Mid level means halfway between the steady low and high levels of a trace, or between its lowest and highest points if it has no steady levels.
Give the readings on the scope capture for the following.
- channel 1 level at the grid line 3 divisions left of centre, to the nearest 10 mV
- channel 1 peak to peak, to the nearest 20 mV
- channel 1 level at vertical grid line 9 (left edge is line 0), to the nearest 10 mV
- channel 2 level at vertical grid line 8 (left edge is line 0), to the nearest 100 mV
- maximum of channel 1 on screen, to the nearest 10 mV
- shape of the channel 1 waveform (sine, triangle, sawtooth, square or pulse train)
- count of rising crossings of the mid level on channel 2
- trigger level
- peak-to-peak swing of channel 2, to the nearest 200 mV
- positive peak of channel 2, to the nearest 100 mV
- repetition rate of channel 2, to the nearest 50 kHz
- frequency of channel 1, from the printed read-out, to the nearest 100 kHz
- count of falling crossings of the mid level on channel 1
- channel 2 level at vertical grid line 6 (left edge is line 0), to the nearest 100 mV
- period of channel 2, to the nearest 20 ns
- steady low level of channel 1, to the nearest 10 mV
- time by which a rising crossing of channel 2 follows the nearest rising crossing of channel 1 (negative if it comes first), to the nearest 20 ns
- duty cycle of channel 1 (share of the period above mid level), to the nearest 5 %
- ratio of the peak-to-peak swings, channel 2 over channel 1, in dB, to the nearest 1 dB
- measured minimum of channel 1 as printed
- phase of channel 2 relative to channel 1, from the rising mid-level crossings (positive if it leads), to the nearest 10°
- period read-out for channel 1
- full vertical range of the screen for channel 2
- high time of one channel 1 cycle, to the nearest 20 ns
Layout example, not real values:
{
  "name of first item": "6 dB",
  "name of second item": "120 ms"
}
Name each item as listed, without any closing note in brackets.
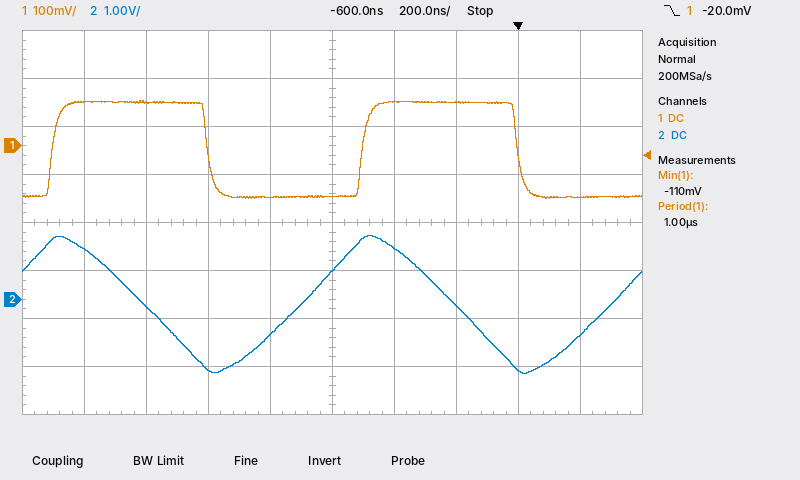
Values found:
{
  "channel 1 level at the grid line 3 divisions left of centre, to the nearest 10 mV": "90 mV",
  "channel 1 peak to peak, to the nearest 20 mV": "200 mV",
  "channel 1 level at vertical grid line 9 (left edge is line 0), to the nearest 10 mV": "-110 mV",
  "channel 2 level at vertical grid line 8 (left edge is line 0), to the nearest 100 mV": "-1.5 V",
  "maximum of channel 1 on screen, to the nearest 10 mV": "90 mV",
  "shape of the channel 1 waveform": "square",
  "count of rising crossings of the mid level on channel 2": "2",
  "trigger level": "-20.0 mV",
  "peak-to-peak swing of channel 2, to the nearest 200 mV": "2.8 V",
  "positive peak of channel 2, to the nearest 100 mV": "1.3 V",
  "repetition rate of channel 2, to the nearest 50 kHz": "1.00 MHz",
  "frequency of channel 1, from the printed read-out, to the nearest 100 kHz": "1.0 MHz",
  "count of falling crossings of the mid level on channel 1": "2",
  "channel 2 level at vertical grid line 6 (left edge is line 0), to the nearest 100 mV": "1.1 V",
  "period of channel 2, to the nearest 20 ns": "1.00 µs",
  "steady low level of channel 1, to the nearest 10 mV": "-110 mV",
  "time by which a rising crossing of channel 2 follows the nearest rising crossing of channel 1 (negative if it comes first), to the nearest 20 ns": "-200 ns",
  "duty cycle of channel 1 (share of the period above mid level), to the nearest 5 %": "50 %",
  "ratio of the peak-to-peak swings, channel 2 over channel 1, in dB, to the nearest 1 dB": "23 dB",
  "measured minimum of channel 1 as printed": "-110 mV",
  "phase of channel 2 relative to channel 1, from the rising mid-level crossings (positive if it leads), to the nearest 10°": "+70°",
  "period read-out for channel 1": "1.00 µs",
  "full vertical range of the screen for channel 2": "8 V",
  "high time of one channel 1 cycle, to the nearest 20 ns": "500 ns"
}
